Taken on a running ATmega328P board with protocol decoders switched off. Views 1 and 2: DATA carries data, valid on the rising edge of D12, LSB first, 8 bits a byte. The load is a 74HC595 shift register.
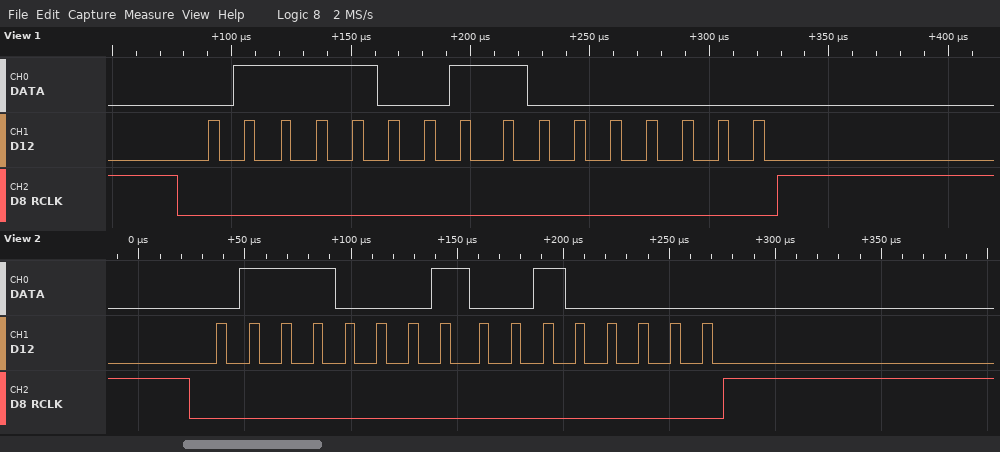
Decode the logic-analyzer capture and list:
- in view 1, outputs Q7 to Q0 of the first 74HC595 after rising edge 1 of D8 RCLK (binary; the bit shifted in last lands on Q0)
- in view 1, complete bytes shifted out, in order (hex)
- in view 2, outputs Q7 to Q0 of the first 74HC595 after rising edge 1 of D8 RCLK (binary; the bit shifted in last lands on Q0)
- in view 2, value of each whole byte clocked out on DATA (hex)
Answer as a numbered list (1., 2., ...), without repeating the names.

1. 10000000
2. 9E 01
3. 00100000
4. 8E 04
